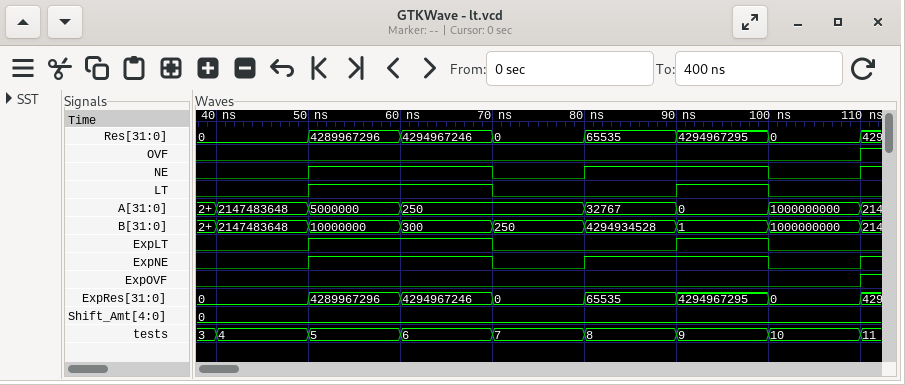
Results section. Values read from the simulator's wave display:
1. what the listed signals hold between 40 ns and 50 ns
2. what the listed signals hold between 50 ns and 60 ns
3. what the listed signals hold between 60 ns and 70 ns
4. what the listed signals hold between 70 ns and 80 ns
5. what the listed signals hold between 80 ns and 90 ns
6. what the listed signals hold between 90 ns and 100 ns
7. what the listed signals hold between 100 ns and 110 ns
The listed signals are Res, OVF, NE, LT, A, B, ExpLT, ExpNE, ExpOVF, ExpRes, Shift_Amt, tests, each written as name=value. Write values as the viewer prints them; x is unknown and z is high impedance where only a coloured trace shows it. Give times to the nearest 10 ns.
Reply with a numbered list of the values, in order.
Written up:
1. Res=0, OVF=0, NE=0, LT=0, A=2147483648, B=2147483648, ExpLT=0, ExpNE=0, ExpOVF=0, ExpRes=0, Shift_Amt=0, tests=4
2. Res=4289967296, OVF=0, NE=1, LT=1, A=5000000, B=10000000, ExpLT=1, ExpNE=1, ExpOVF=0, ExpRes=4289967296, Shift_Amt=0, tests=5
3. Res=4294967246, OVF=0, NE=1, LT=1, A=250, B=300, ExpLT=1, ExpNE=1, ExpOVF=0, ExpRes=4294967246, Shift_Amt=0, tests=6
4. Res=0, OVF=0, NE=0, LT=0, A=250, B=250, ExpLT=0, ExpNE=0, ExpOVF=0, ExpRes=0, Shift_Amt=0, tests=7
5. Res=65535, OVF=0, NE=1, LT=0, A=32767, B=4294934528, ExpLT=0, ExpNE=1, ExpOVF=0, ExpRes=65535, Shift_Amt=0, tests=8
6. Res=4294967295, OVF=0, NE=1, LT=1, A=0, B=1, ExpLT=1, ExpNE=1, ExpOVF=0, ExpRes=4294967295, Shift_Amt=0, tests=9
7. Res=0, OVF=0, NE=0, LT=0, A=1000000000, B=1000000000, ExpLT=0, ExpNE=0, ExpOVF=0, ExpRes=0, Shift_Amt=0, tests=10
